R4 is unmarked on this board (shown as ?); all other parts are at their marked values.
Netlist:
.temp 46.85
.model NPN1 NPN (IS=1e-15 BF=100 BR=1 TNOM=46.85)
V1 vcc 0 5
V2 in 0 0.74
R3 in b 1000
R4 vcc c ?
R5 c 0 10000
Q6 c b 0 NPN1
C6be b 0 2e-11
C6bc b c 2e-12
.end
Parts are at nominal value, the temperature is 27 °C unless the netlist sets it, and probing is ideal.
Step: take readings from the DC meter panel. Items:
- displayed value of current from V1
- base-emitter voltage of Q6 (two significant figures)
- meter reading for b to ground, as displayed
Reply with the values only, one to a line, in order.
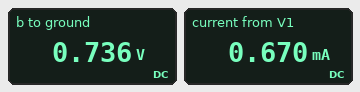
0.670 mA
740 mV
0.736 V
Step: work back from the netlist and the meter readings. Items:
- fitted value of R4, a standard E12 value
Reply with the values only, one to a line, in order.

3.3 kΩ
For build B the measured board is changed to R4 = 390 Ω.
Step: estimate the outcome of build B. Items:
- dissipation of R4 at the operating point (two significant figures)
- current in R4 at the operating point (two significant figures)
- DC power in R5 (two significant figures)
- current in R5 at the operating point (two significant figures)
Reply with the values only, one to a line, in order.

290 µW
860 µA
2.2 mW
470 µA
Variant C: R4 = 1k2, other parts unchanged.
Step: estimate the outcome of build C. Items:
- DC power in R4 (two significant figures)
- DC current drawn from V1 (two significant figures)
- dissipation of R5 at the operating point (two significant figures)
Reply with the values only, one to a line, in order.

760 µW
800 µA
1.6 mW
